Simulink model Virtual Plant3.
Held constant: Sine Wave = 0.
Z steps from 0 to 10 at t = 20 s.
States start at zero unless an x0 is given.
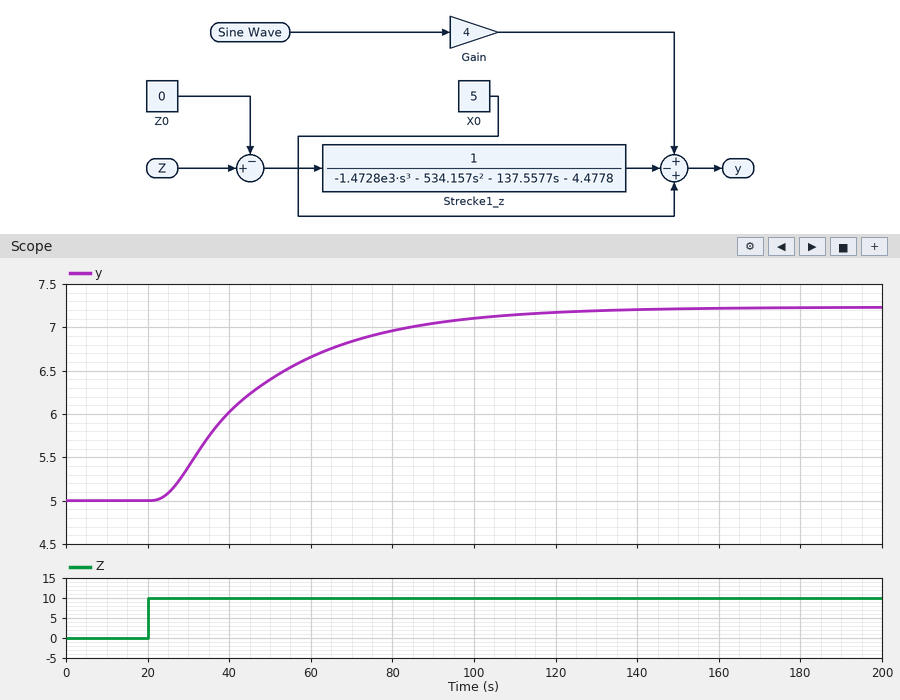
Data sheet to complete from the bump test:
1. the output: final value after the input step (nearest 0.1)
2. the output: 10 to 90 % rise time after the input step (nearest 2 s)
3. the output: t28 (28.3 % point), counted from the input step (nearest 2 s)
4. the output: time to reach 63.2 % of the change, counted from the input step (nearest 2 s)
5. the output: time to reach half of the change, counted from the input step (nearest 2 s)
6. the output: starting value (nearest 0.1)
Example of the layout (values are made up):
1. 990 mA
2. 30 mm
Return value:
1. 7.2
2. 58 s
3. 14 s
4. 30 s
5. 22 s
6. 5.0
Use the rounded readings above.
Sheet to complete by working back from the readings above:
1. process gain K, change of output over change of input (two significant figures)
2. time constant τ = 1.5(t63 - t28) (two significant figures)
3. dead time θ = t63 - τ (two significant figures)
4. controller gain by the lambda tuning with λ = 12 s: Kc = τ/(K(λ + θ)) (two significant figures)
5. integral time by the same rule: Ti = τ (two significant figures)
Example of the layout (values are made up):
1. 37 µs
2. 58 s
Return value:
1. 0.22
2. 24 s
3. 6.0 s
4. 6.1
5. 24 s
